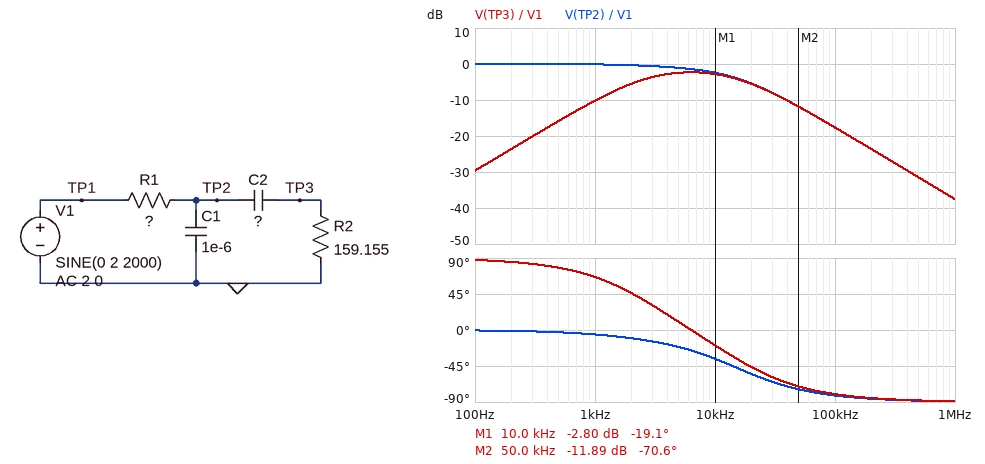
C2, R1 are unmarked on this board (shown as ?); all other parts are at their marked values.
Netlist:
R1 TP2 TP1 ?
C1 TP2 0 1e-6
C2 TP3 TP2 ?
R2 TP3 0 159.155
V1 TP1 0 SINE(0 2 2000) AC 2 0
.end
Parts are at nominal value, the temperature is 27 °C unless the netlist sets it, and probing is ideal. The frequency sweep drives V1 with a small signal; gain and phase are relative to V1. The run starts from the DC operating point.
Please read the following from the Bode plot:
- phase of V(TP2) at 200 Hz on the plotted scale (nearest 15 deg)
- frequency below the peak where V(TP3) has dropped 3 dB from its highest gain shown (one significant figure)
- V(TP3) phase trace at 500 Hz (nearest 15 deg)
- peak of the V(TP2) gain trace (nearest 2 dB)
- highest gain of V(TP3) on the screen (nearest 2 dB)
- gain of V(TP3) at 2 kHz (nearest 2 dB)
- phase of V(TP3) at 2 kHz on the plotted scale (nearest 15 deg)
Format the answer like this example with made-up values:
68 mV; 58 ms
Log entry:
0 deg; 2 kHz; 75 deg; 0 dB; -2 dB; -6 dB; 45 deg
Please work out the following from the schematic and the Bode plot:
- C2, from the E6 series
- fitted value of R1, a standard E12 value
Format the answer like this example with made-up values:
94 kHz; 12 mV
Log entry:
330 nF; 12 Ω
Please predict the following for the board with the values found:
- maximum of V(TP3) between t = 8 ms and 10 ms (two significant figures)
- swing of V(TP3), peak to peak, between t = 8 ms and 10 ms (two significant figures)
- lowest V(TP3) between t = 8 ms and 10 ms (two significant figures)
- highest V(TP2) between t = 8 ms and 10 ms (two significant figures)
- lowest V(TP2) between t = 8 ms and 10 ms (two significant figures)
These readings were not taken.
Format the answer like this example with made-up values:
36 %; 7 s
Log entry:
1.1 V; 2.1 V; -1.1 V; 1.9 V; -1.9 V
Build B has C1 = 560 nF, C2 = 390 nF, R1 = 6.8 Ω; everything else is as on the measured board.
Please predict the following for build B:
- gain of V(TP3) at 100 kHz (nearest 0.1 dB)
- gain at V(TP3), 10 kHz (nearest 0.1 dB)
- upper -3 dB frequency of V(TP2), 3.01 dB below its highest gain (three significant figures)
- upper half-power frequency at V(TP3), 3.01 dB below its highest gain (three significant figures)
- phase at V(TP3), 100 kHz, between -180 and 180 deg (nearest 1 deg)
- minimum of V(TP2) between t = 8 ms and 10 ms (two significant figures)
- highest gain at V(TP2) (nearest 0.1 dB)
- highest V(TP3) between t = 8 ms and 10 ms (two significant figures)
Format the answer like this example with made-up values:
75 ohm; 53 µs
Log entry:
-8.3 dB; -0.9 dB; 39.8 kHz; 48.4 kHz; -65 deg; -2.0 V; 0 dB; 1.2 V
